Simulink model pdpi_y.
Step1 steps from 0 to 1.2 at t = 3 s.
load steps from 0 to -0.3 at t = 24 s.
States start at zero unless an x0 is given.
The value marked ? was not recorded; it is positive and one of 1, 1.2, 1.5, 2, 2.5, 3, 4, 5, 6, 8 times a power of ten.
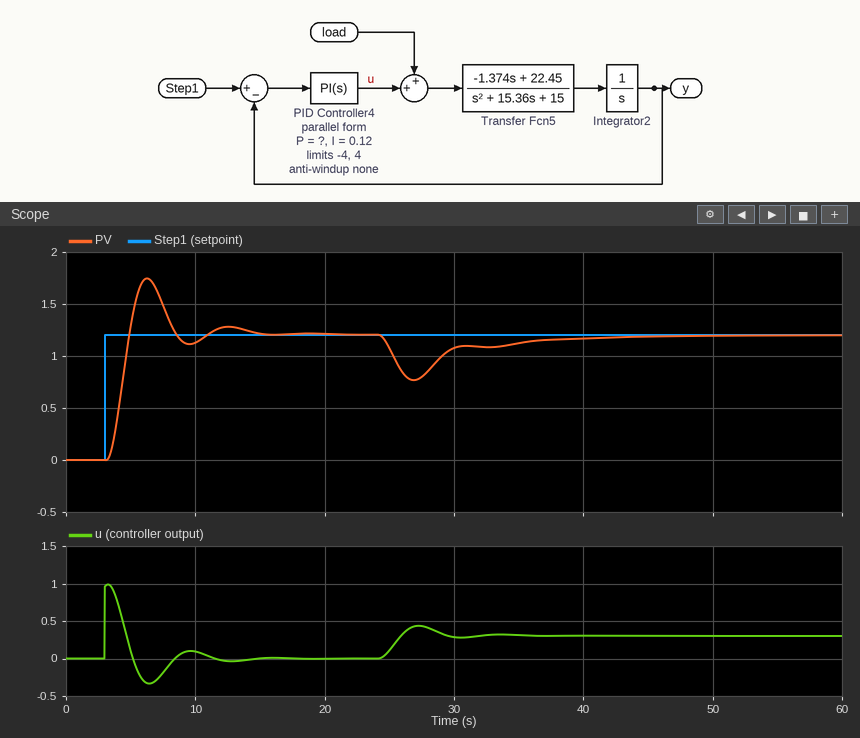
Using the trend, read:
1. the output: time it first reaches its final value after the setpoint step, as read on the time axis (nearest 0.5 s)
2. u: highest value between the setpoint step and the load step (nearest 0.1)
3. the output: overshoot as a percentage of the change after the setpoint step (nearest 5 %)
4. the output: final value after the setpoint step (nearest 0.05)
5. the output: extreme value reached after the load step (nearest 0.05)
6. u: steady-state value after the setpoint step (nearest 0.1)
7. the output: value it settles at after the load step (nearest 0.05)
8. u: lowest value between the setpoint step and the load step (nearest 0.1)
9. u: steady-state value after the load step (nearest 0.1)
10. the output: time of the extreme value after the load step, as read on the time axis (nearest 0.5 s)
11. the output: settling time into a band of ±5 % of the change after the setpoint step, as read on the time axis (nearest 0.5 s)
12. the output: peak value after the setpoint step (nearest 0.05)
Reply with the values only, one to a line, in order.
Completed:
5.0 s
1.0
45 %
1.20
0.75
0.0
1.20
-0.3
0.3
27.0 s
13.5 s
1.75
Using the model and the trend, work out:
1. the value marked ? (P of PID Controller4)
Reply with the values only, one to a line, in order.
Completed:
0.8
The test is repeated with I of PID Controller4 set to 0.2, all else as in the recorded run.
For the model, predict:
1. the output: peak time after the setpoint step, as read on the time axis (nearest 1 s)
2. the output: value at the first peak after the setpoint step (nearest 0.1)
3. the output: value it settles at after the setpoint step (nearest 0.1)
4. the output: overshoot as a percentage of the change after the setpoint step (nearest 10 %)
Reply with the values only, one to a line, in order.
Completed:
6 s
1.9
1.2
60 %
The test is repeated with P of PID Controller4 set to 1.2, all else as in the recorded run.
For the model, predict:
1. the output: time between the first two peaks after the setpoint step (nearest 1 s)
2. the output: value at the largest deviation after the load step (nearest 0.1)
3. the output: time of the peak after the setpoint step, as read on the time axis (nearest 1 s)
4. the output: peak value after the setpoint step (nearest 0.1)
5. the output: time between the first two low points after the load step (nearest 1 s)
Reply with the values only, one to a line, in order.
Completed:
5 s
0.9
6 s
1.8
5 s
